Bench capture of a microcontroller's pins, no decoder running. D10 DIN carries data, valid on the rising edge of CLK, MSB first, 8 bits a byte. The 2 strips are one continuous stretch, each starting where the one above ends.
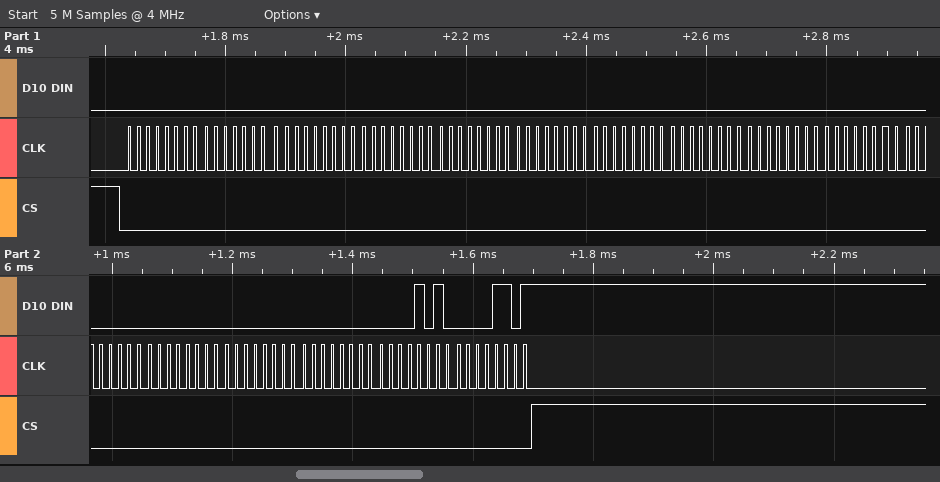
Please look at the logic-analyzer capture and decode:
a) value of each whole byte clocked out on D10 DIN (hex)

00 00 00 00 00 00 00 00 00 00 00 00 00 00 0A 0D
